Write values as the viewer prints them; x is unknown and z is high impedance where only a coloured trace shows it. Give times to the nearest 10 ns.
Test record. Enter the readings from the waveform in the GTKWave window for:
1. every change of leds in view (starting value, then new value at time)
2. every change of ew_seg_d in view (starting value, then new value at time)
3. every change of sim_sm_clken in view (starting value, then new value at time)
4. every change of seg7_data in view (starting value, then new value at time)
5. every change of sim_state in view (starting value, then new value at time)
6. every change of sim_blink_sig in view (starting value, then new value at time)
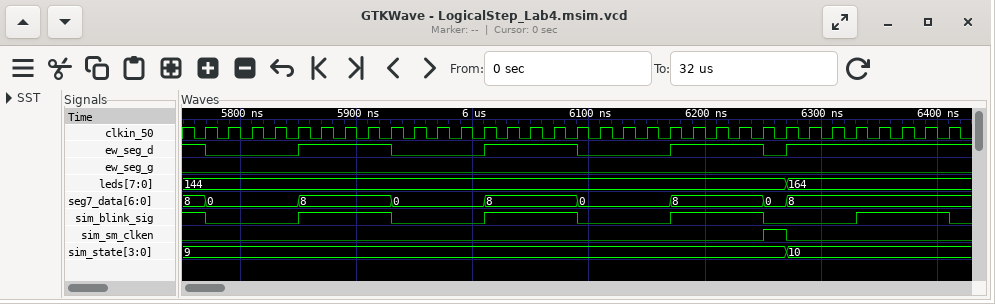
144, 164 at 6270 ns
1, 0 at 5770 ns, 1 at 5850 ns, 0 at 5930 ns, 1 at 6010 ns, 0 at 6090 ns, 1 at 6170 ns, 0 at 6250 ns, 1 at 6270 ns
0, 1 at 6250 ns, 0 at 6270 ns
8, 0 at 5770 ns, 8 at 5850 ns, 0 at 5930 ns, 8 at 6010 ns, 0 at 6090 ns, 8 at 6170 ns, 0 at 6250 ns, 8 at 6270 ns
9, 10 at 6270 ns
1, 0 at 5770 ns, 1 at 5850 ns, 0 at 5930 ns, 1 at 6010 ns, 0 at 6090 ns, 1 at 6170 ns, 0 at 6250 ns, 1 at 6330 ns, 0 at 6410 ns
